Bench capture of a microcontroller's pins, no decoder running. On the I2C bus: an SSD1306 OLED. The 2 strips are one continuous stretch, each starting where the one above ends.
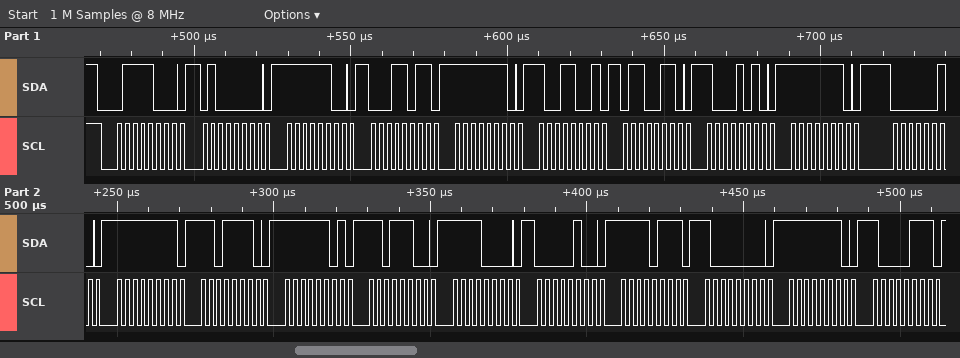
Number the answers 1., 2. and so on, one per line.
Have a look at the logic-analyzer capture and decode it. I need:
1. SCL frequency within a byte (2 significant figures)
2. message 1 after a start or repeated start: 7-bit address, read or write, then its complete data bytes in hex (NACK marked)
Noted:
1. 400 kHz
2. 0x3C write: 40 FC 1B FE 99 66 8A FE 02 FF DE FD DC F0 04 F7 80 FE 87
